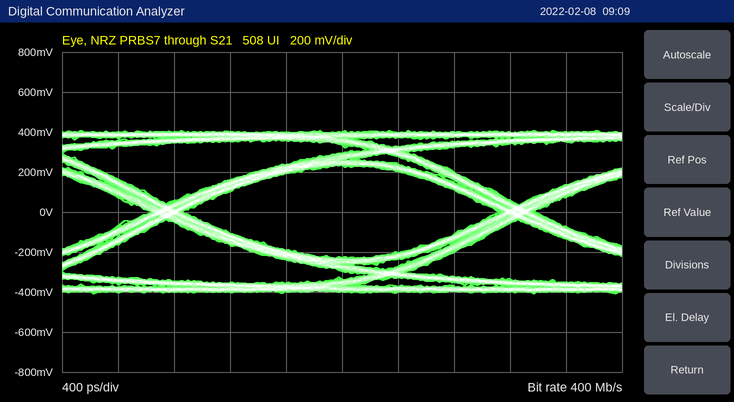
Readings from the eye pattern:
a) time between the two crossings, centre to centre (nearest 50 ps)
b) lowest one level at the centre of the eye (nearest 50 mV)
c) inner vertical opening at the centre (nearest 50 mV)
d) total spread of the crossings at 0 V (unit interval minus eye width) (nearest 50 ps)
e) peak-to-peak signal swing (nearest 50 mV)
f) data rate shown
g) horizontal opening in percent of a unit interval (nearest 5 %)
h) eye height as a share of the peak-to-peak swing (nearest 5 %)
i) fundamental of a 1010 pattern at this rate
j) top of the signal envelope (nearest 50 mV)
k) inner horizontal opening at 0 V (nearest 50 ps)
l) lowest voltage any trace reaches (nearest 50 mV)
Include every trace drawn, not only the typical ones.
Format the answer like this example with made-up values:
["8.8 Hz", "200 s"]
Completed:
["2.50 ns", "250 mV", "450 mV", "250 ps", "800 mV", "400 Mb/s", "90 %", "55 %", "200 MHz", "400 mV", "2.25 ns", "-400 mV"]
